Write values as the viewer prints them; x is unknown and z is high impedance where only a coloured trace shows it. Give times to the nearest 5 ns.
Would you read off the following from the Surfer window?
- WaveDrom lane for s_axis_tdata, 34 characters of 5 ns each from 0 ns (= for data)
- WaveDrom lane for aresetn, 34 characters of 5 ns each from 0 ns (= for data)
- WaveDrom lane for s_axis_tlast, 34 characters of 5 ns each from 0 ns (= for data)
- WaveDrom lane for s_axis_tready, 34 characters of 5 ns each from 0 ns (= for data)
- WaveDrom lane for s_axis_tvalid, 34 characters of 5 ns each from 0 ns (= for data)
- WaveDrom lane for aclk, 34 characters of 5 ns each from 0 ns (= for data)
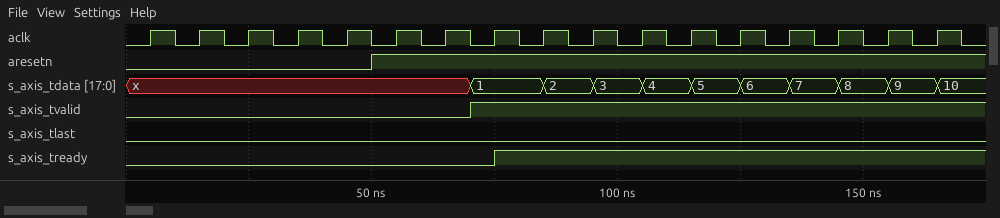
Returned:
{name: 's_axis_tdata', wave: 'x.............=..=.=.=.=.=.=.=.=.=', data: '1 2 3 4 5 6 7 8 9 10'}
{name: 'aresetn', wave: '0.........1.......................'}
{name: 's_axis_tlast', wave: '0.................................'}
{name: 's_axis_tready', wave: '0..............1..................'}
{name: 's_axis_tvalid', wave: '0.............1...................'}
{name: 'aclk', wave: '0101010101010101010101010101010101'}
